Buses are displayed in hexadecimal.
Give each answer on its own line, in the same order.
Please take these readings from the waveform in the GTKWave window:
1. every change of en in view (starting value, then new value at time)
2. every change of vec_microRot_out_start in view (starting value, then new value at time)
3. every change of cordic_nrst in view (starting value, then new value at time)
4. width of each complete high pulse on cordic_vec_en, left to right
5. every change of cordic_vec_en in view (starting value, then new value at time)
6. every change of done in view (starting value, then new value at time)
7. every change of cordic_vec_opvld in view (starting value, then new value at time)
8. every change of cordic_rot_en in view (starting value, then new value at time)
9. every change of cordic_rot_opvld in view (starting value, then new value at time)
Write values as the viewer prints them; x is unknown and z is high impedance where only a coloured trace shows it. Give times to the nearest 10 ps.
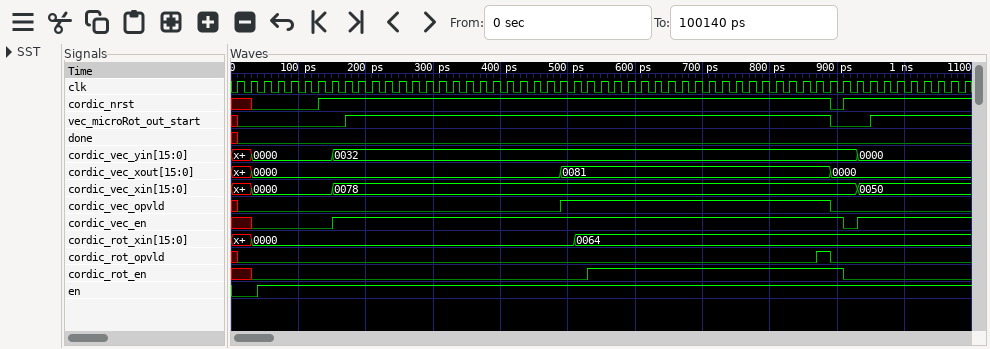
0, 1 at 40 ps
x, 0 at 10 ps, 1 at 170 ps, 0 at 890 ps, 1 at 950 ps
x, 0 at 30 ps, 1 at 130 ps, 0 at 890 ps, 1 at 910 ps
760 ps
x, 0 at 30 ps, 1 at 150 ps, 0 at 910 ps, 1 at 930 ps
x, 0 at 10 ps
x, 0 at 10 ps, 1 at 490 ps, 0 at 890 ps
x, 0 at 30 ps, 1 at 530 ps, 0 at 910 ps
x, 0 at 10 ps, 1 at 870 ps, 0 at 890 ps
